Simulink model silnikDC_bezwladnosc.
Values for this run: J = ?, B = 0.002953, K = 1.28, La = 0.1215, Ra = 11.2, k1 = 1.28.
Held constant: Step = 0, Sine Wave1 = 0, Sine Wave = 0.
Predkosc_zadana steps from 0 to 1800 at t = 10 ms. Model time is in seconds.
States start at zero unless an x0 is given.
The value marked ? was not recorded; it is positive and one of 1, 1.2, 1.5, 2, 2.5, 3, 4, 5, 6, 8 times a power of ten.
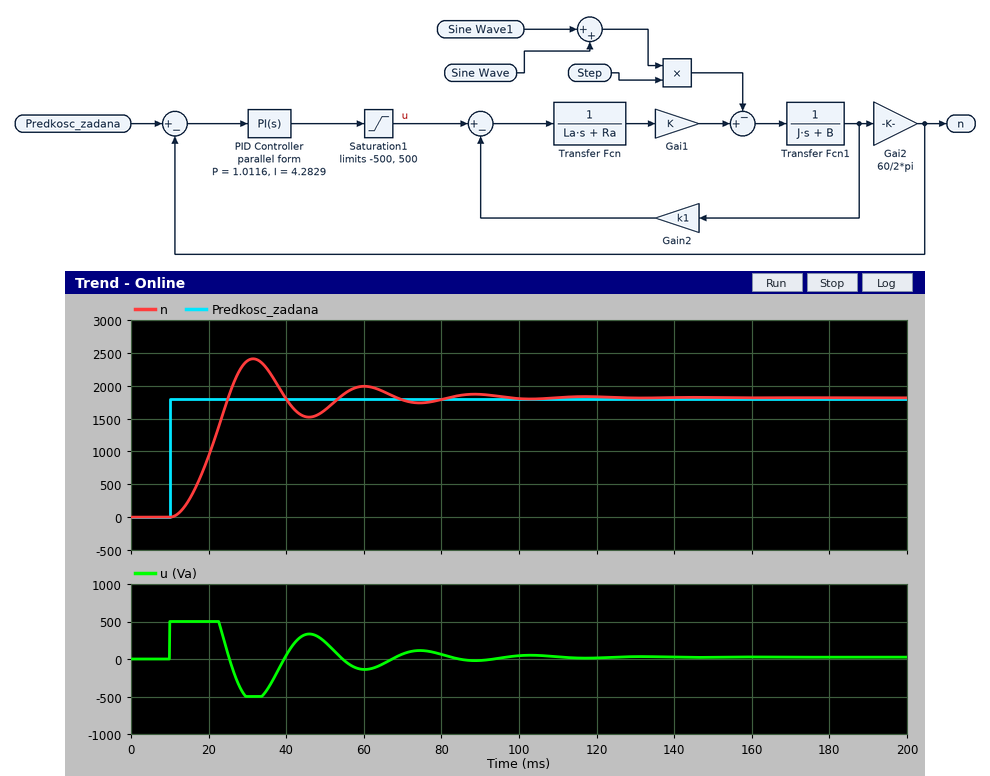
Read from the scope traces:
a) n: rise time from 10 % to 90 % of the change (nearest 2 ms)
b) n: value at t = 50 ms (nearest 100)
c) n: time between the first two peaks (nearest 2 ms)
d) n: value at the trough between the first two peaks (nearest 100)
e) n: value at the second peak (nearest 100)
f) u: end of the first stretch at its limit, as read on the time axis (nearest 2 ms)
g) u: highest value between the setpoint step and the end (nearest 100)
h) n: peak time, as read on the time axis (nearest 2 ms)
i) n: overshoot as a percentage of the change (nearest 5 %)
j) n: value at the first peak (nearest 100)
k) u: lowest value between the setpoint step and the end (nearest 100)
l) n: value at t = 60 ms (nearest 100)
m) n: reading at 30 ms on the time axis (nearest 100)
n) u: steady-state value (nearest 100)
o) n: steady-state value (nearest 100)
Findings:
10 ms
1600
28 ms
1500
2000
22 ms
500
32 ms
35 %
2400
-500
2000
2400
0
1800
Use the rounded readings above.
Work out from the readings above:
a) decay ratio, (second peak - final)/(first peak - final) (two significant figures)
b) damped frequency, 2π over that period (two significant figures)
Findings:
0.33
0.22 rad/ms
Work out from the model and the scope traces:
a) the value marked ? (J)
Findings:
0.02
